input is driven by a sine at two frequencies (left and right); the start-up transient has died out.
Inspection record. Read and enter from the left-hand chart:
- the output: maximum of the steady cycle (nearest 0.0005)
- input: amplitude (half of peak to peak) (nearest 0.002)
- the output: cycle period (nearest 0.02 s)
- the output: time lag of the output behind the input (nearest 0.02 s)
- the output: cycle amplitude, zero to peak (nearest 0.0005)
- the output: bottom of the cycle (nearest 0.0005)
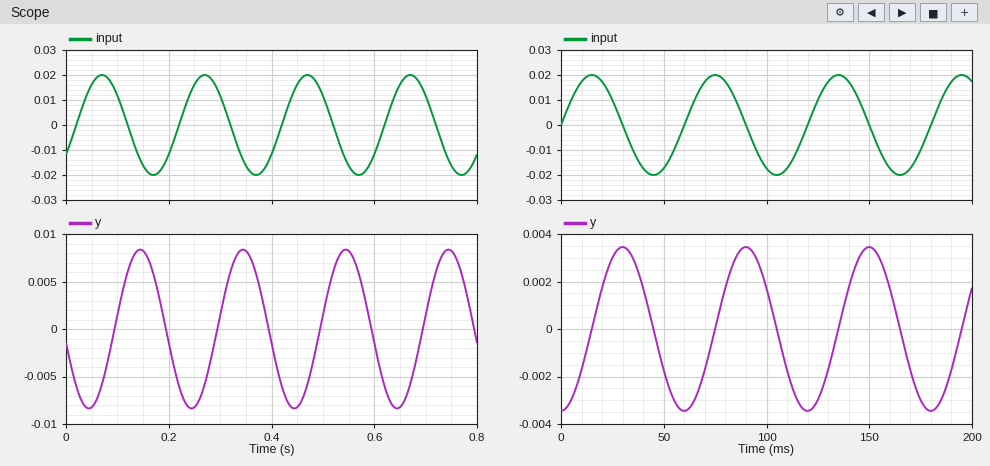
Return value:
0.0085
0.020
0.20 s
0.08 s
0.0085
-0.0085
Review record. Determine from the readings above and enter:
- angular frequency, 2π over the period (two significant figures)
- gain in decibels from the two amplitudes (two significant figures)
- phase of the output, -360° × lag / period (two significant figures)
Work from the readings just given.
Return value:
31 rad/s
-7.4 dB
-140°
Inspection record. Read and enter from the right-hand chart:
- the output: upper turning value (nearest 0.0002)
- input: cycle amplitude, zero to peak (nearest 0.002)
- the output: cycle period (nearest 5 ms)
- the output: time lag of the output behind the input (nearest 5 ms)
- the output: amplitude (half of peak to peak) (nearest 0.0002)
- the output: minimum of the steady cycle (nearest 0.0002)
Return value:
0.0034
0.020
60 ms
15 ms
0.0034
-0.0034
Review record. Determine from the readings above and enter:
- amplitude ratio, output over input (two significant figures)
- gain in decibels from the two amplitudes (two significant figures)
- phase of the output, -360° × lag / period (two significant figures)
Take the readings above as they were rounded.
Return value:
0.17
-15 dB
-90°
